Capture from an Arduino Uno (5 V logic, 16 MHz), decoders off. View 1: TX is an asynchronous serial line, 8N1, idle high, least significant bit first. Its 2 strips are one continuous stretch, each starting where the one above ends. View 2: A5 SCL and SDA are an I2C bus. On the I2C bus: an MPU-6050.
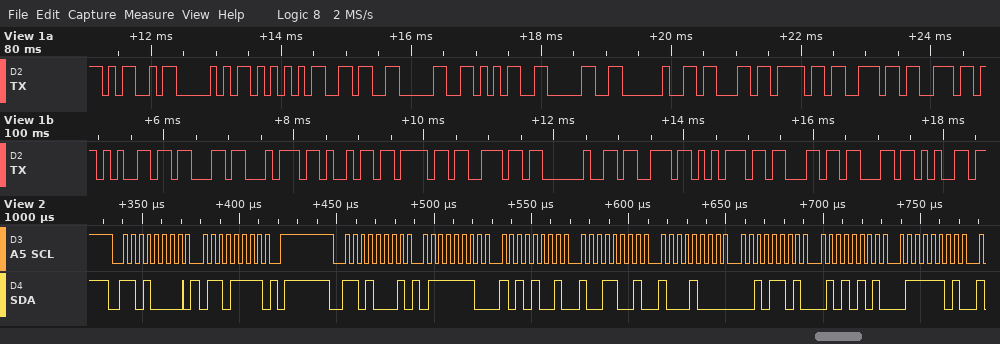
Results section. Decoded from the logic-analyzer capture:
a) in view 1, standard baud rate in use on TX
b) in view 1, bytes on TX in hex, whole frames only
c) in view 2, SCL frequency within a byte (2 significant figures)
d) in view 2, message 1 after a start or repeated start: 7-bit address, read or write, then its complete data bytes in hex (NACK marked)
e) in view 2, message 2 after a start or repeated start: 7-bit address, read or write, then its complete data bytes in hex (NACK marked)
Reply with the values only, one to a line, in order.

9600 baud
0x4D 0x50 0x55 0x36 0x30 0x35 0x30 0x20 0x63 0x6F 0x6E 0x6E 0x65 0x63 0x74 0x69 0x6F 0x6E 0x20 0x73 0x75 0x63 0x63 0x65
250 kHz
0x68 write: 6F
0x68 read: 7E A9 99 88 2D 55 7D
